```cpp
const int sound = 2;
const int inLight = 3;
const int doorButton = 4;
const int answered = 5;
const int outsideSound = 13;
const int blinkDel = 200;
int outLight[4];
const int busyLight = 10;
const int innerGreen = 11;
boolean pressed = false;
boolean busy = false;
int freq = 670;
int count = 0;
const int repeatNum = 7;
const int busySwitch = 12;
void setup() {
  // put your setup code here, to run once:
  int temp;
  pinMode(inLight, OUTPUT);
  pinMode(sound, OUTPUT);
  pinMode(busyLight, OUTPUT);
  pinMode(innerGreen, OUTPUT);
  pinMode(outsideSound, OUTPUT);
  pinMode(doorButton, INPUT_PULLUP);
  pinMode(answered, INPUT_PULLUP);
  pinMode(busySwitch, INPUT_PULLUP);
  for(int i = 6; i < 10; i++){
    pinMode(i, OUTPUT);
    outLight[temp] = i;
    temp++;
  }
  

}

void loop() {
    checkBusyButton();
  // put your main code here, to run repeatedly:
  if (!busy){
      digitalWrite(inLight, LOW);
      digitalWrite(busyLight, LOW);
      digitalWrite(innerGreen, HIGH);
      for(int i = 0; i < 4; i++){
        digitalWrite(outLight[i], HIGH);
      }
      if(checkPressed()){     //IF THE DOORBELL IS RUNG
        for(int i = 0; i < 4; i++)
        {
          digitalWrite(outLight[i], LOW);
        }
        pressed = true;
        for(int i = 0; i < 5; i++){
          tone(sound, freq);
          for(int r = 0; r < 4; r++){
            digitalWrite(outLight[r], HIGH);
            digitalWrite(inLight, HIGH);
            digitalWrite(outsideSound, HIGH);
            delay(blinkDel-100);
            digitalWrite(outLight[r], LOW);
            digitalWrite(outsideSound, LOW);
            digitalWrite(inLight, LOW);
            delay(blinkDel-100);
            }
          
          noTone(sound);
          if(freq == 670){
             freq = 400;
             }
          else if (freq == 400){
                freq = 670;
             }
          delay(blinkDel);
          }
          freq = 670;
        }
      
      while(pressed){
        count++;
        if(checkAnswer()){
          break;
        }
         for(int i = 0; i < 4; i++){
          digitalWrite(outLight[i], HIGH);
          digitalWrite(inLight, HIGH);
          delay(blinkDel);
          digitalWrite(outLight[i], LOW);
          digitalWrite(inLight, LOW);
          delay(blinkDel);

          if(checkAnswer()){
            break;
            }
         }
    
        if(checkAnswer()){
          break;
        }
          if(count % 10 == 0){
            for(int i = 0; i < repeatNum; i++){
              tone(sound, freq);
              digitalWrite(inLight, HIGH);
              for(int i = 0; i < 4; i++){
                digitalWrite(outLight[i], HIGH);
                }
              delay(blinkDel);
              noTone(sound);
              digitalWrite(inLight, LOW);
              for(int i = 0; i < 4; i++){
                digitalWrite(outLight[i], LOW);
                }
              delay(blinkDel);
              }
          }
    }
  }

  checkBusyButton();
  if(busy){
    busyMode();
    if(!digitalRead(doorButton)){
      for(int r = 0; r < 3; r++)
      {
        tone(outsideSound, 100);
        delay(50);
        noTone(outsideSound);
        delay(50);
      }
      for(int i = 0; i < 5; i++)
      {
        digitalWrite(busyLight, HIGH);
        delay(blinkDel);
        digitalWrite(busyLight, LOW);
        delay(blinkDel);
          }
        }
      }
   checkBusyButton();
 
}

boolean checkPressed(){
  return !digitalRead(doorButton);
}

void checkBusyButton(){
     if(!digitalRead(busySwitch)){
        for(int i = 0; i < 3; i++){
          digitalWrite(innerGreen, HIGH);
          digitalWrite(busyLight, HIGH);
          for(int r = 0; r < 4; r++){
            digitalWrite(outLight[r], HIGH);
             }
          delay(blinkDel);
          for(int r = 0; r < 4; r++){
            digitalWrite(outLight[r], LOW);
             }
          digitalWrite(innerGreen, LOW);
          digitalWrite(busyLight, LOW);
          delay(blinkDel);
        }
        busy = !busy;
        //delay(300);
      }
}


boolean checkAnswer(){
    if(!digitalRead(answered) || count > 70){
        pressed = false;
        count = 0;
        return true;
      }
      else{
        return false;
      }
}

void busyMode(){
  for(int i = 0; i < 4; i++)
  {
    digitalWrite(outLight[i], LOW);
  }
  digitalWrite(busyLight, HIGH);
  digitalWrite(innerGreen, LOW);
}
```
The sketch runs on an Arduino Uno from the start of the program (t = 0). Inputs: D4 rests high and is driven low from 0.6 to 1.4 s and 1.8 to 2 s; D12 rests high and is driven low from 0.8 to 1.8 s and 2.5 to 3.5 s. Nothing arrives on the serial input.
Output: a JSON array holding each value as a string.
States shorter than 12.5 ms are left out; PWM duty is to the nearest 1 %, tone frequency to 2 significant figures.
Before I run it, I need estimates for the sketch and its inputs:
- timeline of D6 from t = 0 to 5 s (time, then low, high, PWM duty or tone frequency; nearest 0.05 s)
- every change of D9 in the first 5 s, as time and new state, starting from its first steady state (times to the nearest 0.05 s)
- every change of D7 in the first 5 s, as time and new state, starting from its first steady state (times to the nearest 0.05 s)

["0 s high; 0.7 s low; 1.6 s high; 1.7 s low; 2.6 s high; 2.7 s low; 3.6 s high; 3.7 s low; 4.6 s high; 4.7 s low", "0 s high; 0.6 s low; 1.2 s high; 1.3 s low; 2.2 s high; 2.3 s low; 3.2 s high; 3.3 s low; 4.2 s high; 4.3 s low", "0 s high; 0.6 s low; 0.8 s high; 0.9 s low; 1.8 s high; 1.9 s low; 2.8 s high; 2.9 s low; 3.8 s high; 3.9 s low; 4.8 s high; 4.9 s low"]
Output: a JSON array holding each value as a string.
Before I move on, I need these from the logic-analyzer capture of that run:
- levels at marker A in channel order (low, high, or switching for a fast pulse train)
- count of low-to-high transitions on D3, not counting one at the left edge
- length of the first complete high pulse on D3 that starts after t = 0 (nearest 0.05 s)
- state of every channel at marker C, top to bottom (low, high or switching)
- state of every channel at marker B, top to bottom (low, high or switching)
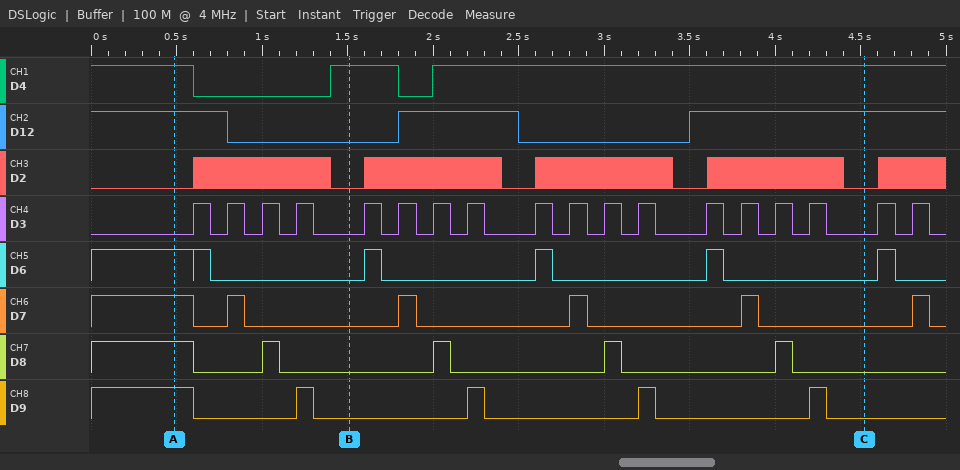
["D4 high, D12 high, D2 low, D3 low, D6 high, D7 high, D8 high, D9 high", "18", "0.10 s", "D4 high, D12 high, D2 low, D3 low, D6 low, D7 low, D8 low, D9 low", "D4 high, D12 low, D2 low, D3 low, D6 low, D7 low, D8 low, D9 low"]
